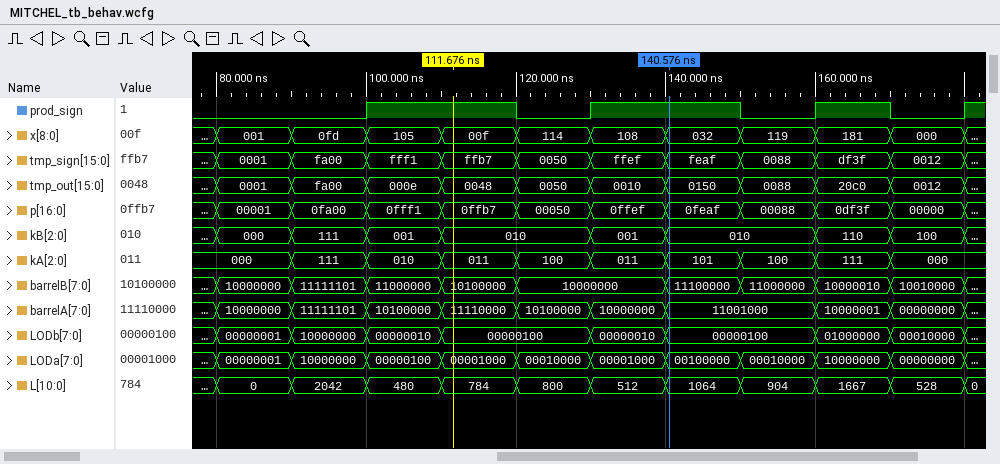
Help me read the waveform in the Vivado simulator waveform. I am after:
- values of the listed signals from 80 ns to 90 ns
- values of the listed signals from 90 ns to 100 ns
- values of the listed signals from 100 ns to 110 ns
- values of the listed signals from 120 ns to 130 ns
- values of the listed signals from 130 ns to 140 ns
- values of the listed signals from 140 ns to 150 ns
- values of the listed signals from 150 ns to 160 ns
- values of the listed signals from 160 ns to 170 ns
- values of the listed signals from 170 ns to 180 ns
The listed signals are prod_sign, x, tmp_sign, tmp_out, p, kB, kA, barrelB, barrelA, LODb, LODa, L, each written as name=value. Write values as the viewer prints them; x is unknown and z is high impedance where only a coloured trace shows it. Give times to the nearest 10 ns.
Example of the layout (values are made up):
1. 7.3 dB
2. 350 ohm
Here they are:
1. prod_sign=0, x=001, tmp_sign=0001, tmp_out=0001, p=00001, kB=000, kA=000, barrelB=10000000, barrelA=10000000, LODb=00000001, LODa=00000001, L=0
2. prod_sign=0, x=0fd, tmp_sign=fa00, tmp_out=fa00, p=0fa00, kB=111, kA=111, barrelB=11111101, barrelA=11111101, LODb=10000000, LODa=10000000, L=2042
3. prod_sign=1, x=105, tmp_sign=fff1, tmp_out=000e, p=0fff1, kB=001, kA=010, barrelB=11000000, barrelA=10100000, LODb=00000010, LODa=00000100, L=480
4. prod_sign=0, x=114, tmp_sign=0050, tmp_out=0050, p=00050, kB=010, kA=100, barrelB=10000000, barrelA=10100000, LODb=00000100, LODa=00010000, L=800
5. prod_sign=1, x=108, tmp_sign=ffef, tmp_out=0010, p=0ffef, kB=001, kA=011, barrelB=10000000, barrelA=10000000, LODb=00000010, LODa=00001000, L=512
6. prod_sign=1, x=032, tmp_sign=feaf, tmp_out=0150, p=0feaf, kB=010, kA=101, barrelB=11100000, barrelA=11001000, LODb=00000100, LODa=00100000, L=1064
7. prod_sign=0, x=119, tmp_sign=0088, tmp_out=0088, p=00088, kB=010, kA=100, barrelB=11000000, barrelA=11001000, LODb=00000100, LODa=00010000, L=904
8. prod_sign=1, x=181, tmp_sign=df3f, tmp_out=20c0, p=0df3f, kB=110, kA=111, barrelB=10000010, barrelA=10000001, LODb=01000000, LODa=10000000, L=1667
9. prod_sign=0, x=000, tmp_sign=0012, tmp_out=0012, p=00000, kB=100, kA=000, barrelB=10010000, barrelA=00000000, LODb=00010000, LODa=00000000, L=528
